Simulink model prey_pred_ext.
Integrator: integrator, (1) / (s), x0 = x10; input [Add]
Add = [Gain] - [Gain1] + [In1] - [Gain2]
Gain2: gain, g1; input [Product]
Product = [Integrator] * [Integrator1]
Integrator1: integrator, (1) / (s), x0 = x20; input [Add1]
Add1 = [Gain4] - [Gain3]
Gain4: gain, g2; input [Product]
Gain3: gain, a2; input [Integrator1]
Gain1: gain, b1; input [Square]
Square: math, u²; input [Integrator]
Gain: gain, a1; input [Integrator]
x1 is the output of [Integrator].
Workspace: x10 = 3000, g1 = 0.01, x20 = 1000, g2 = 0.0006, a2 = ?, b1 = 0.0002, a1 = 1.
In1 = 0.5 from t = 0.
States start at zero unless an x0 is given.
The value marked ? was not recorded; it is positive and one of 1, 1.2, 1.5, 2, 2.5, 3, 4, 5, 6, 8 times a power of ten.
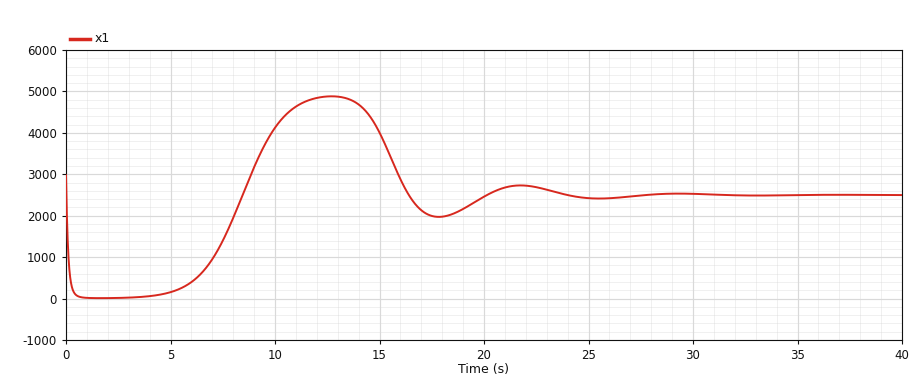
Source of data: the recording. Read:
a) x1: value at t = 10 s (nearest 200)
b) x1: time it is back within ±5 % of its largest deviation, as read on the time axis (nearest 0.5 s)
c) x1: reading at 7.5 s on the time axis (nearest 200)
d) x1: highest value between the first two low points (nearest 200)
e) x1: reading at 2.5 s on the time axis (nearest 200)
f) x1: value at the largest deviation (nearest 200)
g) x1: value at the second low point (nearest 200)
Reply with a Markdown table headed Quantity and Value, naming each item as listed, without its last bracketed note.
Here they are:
| Quantity | Value |
|---|---|
| x1: value at t = 10 s | 4200 |
| x1: time it is back within ±5 % of its largest deviation, as read on the time axis | 23.0 s |
| x1: reading at 7.5 s on the time axis | 1400 |
| x1: highest value between the first two low points | 4800 |
| x1: reading at 2.5 s on the time axis | 0 |
| x1: value at the largest deviation | 0 |
| x1: value at the second low point | 2000 |
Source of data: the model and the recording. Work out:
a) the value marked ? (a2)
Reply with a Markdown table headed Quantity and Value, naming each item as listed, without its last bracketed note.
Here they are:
| Quantity | Value |
|---|---|
| the value marked ? | 1.5 |
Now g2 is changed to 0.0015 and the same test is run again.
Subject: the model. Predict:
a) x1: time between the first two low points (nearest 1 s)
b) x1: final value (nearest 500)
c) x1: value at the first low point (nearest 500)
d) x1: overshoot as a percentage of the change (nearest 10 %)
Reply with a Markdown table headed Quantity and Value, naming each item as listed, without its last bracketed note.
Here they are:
| Quantity | Value |
|---|---|
| x1: time between the first two low points | 12 s |
| x1: final value | 1000 |
| x1: value at the first low point | 0 |
| x1: overshoot as a percentage of the change | 50 % |
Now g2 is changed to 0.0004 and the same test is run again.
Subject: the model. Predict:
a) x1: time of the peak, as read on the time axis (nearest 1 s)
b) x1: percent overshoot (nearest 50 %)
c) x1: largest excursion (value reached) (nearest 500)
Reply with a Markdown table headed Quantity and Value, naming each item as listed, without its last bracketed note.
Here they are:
| Quantity | Value |
|---|---|
| x1: time of the peak, as read on the time axis | 15 s |
| x1: percent overshoot | 150 % |
| x1: largest excursion (value reached) | 5000 |
